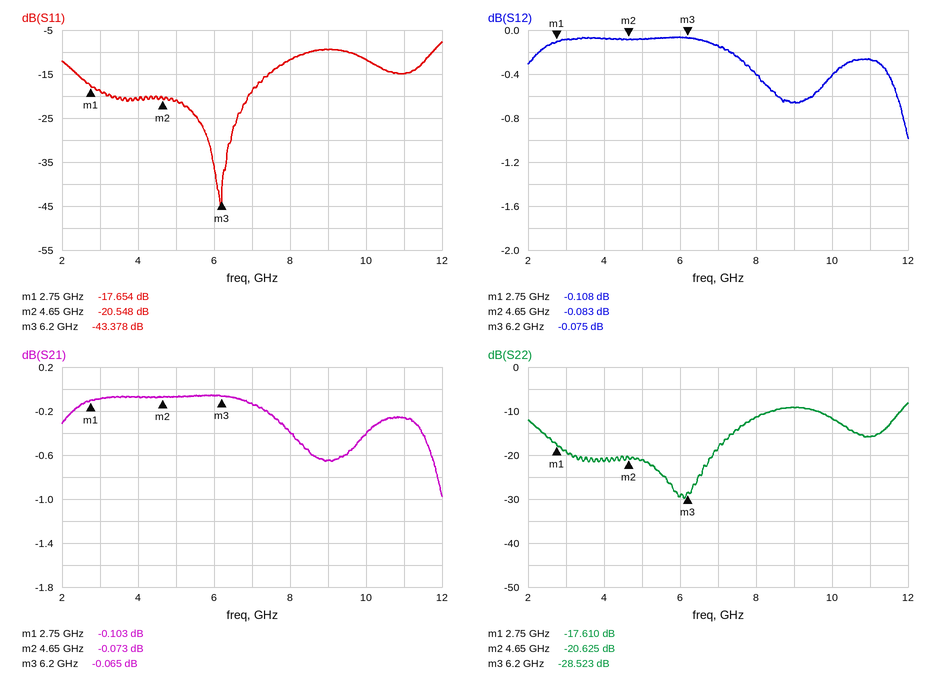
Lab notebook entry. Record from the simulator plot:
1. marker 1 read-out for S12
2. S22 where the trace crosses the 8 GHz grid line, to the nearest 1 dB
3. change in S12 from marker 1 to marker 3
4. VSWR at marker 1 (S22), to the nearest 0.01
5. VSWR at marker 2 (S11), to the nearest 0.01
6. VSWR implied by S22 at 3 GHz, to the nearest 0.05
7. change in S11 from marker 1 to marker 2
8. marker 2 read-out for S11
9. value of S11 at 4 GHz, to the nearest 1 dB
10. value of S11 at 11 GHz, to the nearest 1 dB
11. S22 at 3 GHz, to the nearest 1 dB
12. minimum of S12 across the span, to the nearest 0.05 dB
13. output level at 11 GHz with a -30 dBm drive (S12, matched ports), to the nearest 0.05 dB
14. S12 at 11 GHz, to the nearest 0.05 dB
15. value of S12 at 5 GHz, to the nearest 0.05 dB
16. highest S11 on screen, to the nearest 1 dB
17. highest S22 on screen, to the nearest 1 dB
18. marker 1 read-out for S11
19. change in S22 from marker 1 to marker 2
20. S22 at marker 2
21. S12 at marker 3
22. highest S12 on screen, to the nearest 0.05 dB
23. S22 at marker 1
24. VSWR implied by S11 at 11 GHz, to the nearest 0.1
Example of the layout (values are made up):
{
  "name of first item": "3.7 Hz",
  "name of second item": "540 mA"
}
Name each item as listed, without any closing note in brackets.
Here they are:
{
  "marker 1 read-out for S12": "-0.108 dB",
  "S22 where the trace crosses the 8 GHz grid line, to the nearest 1 dB": "-11 dB",
  "change in S12 from marker 1 to marker 3": "0.033 dB",
  "VSWR at marker 1 (S22), to the nearest 0.01": "1.30",
  "VSWR at marker 2 (S11), to the nearest 0.01": "1.21",
  "VSWR implied by S22 at 3 GHz, to the nearest 0.05": "1.25",
  "change in S11 from marker 1 to marker 2": "-2.894 dB",
  "marker 2 read-out for S11": "-20.548 dB",
  "value of S11 at 4 GHz, to the nearest 1 dB": "-21 dB",
  "value of S11 at 11 GHz, to the nearest 1 dB": "-15 dB",
  "S22 at 3 GHz, to the nearest 1 dB": "-19 dB",
  "minimum of S12 across the span, to the nearest 0.05 dB": "-1.00 dB",
  "output level at 11 GHz with a -30 dBm drive (S12, matched ports), to the nearest 0.05 dB": "-30.25 dBm",
  "S12 at 11 GHz, to the nearest 0.05 dB": "-0.25 dB",
  "value of S12 at 5 GHz, to the nearest 0.05 dB": "-0.10 dB",
  "highest S11 on screen, to the nearest 1 dB": "-8 dB",
  "highest S22 on screen, to the nearest 1 dB": "-8 dB",
  "marker 1 read-out for S11": "-17.654 dB",
  "change in S22 from marker 1 to marker 2": "-3.015 dB",
  "S22 at marker 2": "-20.625 dB",
  "S12 at marker 3": "-0.075 dB",
  "highest S12 on screen, to the nearest 0.05 dB": "-0.05 dB",
  "S22 at marker 1": "-17.610 dB",
  "VSWR implied by S11 at 11 GHz, to the nearest 0.1": "1.4"
}
